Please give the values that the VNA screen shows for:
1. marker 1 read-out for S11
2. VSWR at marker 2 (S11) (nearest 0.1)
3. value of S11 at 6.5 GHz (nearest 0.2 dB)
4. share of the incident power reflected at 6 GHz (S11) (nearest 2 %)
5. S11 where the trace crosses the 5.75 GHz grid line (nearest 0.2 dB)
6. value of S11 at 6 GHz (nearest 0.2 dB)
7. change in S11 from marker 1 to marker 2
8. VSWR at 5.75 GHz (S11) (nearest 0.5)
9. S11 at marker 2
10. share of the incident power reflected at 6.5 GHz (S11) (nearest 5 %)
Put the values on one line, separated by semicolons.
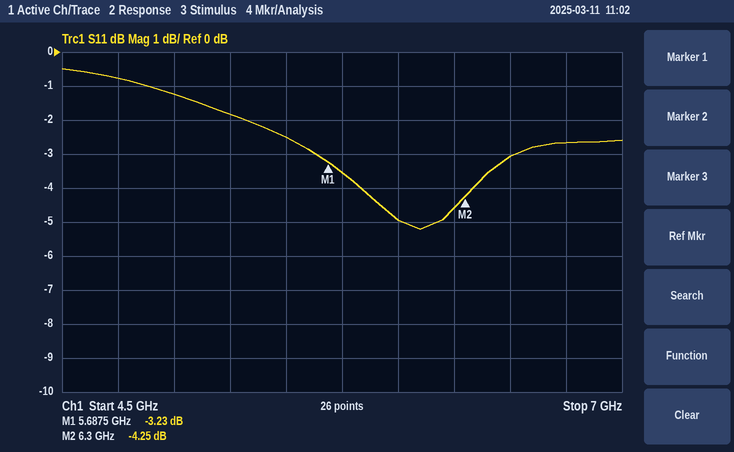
-3.23 dB; 4.2; -3.0 dB; 32 %; -3.6 dB; -5.0 dB; -1.02 dB; 5.0; -4.25 dB; 50 %
